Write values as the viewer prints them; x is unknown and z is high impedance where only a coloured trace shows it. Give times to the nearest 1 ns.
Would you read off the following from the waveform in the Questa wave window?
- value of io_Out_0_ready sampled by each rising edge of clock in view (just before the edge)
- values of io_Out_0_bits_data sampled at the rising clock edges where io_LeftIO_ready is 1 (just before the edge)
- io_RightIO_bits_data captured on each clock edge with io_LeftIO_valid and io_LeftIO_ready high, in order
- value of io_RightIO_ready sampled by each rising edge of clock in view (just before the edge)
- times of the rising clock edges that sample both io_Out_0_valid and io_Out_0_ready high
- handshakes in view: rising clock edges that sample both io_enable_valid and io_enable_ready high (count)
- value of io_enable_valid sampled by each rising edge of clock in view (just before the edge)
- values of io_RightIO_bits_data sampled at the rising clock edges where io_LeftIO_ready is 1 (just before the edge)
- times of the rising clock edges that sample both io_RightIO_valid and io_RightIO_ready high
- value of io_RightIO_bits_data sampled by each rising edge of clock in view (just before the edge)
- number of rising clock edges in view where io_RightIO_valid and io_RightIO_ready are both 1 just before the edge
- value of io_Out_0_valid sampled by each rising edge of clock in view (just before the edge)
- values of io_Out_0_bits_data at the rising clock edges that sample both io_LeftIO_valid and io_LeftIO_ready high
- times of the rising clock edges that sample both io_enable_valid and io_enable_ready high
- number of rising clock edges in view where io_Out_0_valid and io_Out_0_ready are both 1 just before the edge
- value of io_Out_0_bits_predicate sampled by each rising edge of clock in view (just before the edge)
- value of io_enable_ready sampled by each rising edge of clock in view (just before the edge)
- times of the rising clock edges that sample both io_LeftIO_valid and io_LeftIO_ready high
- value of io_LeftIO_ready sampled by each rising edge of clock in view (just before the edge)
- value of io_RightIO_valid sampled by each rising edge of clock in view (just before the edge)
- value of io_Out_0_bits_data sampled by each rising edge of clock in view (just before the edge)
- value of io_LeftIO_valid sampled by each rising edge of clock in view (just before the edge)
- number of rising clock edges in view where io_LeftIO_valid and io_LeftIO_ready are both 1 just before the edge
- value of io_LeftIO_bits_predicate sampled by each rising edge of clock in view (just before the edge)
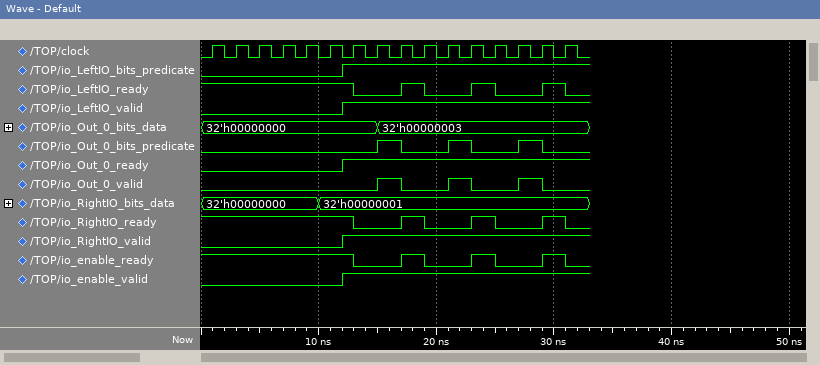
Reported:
0 0 0 0 0 0 1 1 1 1 1 1 1 1 1 1
32'h00000000, 32'h00000000, 32'h00000000, 32'h00000000, 32'h00000000, 32'h00000000, 32'h00000000, 32'h00000003, 32'h00000003, 32'h00000003
32'h00000001, 32'h00000001, 32'h00000001, 32'h00000001
1 1 1 1 1 1 1 0 0 1 0 0 1 0 0 1
17 ns, 23 ns, 29 ns
4
0 0 0 0 0 0 1 1 1 1 1 1 1 1 1 1
32'h00000000, 32'h00000000, 32'h00000000, 32'h00000000, 32'h00000000, 32'h00000001, 32'h00000001, 32'h00000001, 32'h00000001, 32'h00000001
13 ns, 19 ns, 25 ns, 31 ns
32'h00000000, 32'h00000000, 32'h00000000, 32'h00000000, 32'h00000000, 32'h00000001, 32'h00000001, 32'h00000001, 32'h00000001, 32'h00000001, 32'h00000001, 32'h00000001, 32'h00000001, 32'h00000001, 32'h00000001, 32'h00000001
4
0 0 0 0 0 0 0 0 1 0 0 1 0 0 1 0
32'h00000000, 32'h00000003, 32'h00000003, 32'h00000003
13 ns, 19 ns, 25 ns, 31 ns
3
0 0 0 0 0 0 0 0 1 0 0 1 0 0 1 0
1 1 1 1 1 1 1 0 0 1 0 0 1 0 0 1
13 ns, 19 ns, 25 ns, 31 ns
1 1 1 1 1 1 1 0 0 1 0 0 1 0 0 1
0 0 0 0 0 0 1 1 1 1 1 1 1 1 1 1
32'h00000000, 32'h00000000, 32'h00000000, 32'h00000000, 32'h00000000, 32'h00000000, 32'h00000000, 32'h00000000, 32'h00000003, 32'h00000003, 32'h00000003, 32'h00000003, 32'h00000003, 32'h00000003, 32'h00000003, 32'h00000003
0 0 0 0 0 0 1 1 1 1 1 1 1 1 1 1
4
0 0 0 0 0 0 1 1 1 1 1 1 1 1 1 1
